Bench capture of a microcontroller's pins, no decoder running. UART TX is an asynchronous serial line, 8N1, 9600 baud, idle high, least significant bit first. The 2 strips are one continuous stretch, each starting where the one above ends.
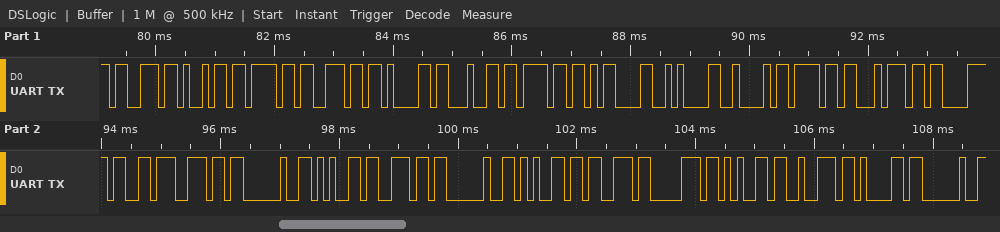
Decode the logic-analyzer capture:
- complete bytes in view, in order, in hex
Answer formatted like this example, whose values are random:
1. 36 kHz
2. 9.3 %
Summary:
1. 73 69 6F 6E 61 64 6F 0D 0A 42 6F 74 C3 B3 6E 20 65 6E 20 65 73 70 65 72 61 20
